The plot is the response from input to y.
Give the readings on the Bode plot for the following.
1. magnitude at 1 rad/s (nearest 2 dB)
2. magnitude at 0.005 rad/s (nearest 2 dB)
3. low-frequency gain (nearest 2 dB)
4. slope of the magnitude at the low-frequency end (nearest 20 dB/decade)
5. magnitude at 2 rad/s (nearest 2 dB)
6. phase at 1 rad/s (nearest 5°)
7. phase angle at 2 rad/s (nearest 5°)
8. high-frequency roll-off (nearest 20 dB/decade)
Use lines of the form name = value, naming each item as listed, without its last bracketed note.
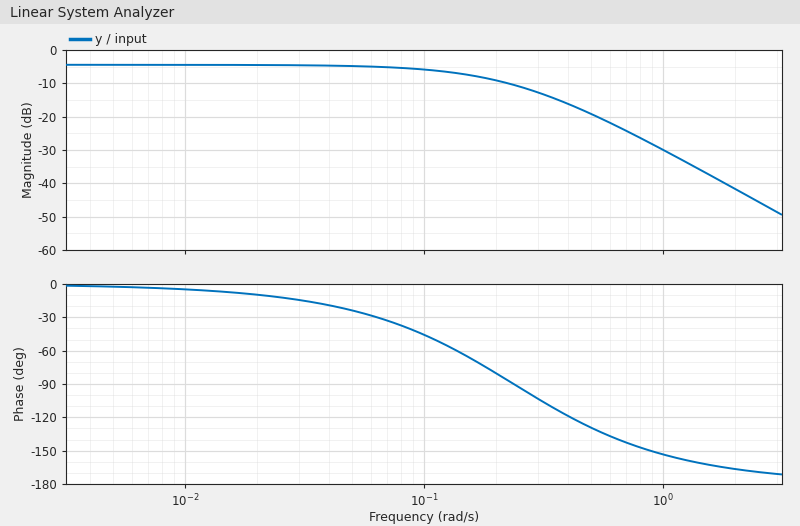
magnitude at 1 rad/s = -30 dB
magnitude at 0.005 rad/s = -4 dB
low-frequency gain = -4 dB
slope of the magnitude at the low-frequency end = 0 dB/decade
magnitude at 2 rad/s = -42 dB
phase at 1 rad/s = -155°
phase angle at 2 rad/s = -165°
high-frequency roll-off = -40 dB/decade
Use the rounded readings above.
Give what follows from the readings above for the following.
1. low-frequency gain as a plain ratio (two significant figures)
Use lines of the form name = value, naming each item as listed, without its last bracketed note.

low-frequency gain as a plain ratio = 0.63
